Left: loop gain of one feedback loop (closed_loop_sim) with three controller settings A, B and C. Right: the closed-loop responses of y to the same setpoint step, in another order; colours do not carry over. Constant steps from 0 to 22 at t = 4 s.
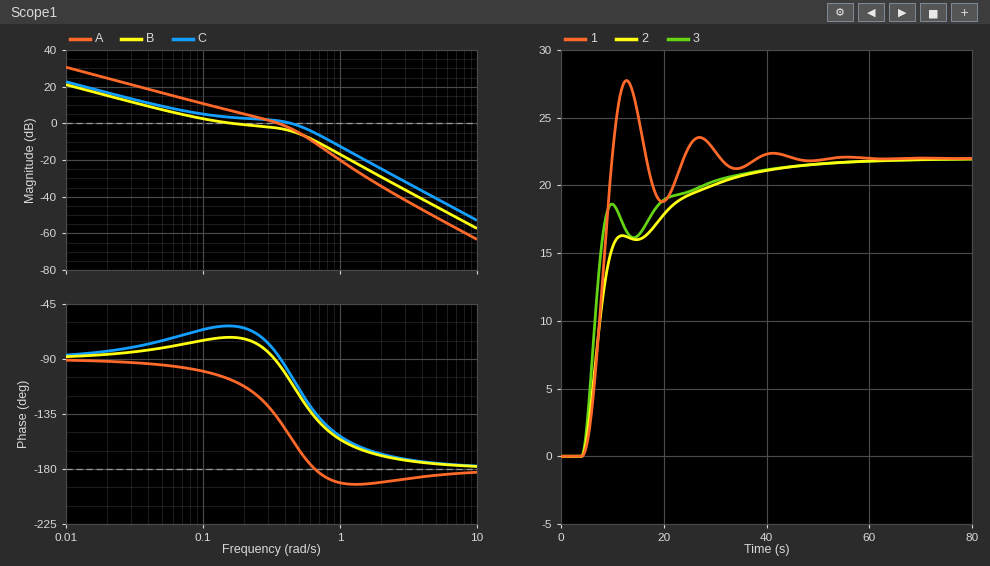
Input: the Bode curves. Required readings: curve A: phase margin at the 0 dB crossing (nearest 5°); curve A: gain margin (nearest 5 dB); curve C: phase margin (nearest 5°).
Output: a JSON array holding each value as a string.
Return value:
["40°", "10 dB", "75°"]
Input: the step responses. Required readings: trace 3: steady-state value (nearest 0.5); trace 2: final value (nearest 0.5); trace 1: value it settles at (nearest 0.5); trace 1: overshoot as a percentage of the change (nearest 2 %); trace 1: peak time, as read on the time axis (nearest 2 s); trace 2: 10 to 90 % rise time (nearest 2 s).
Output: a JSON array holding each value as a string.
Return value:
["22.0", "22.0", "22.0", "26 %", "12 s", "22 s"]
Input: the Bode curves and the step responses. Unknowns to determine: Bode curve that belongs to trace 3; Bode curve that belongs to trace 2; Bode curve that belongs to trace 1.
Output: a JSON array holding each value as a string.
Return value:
["C", "B", "A"]
